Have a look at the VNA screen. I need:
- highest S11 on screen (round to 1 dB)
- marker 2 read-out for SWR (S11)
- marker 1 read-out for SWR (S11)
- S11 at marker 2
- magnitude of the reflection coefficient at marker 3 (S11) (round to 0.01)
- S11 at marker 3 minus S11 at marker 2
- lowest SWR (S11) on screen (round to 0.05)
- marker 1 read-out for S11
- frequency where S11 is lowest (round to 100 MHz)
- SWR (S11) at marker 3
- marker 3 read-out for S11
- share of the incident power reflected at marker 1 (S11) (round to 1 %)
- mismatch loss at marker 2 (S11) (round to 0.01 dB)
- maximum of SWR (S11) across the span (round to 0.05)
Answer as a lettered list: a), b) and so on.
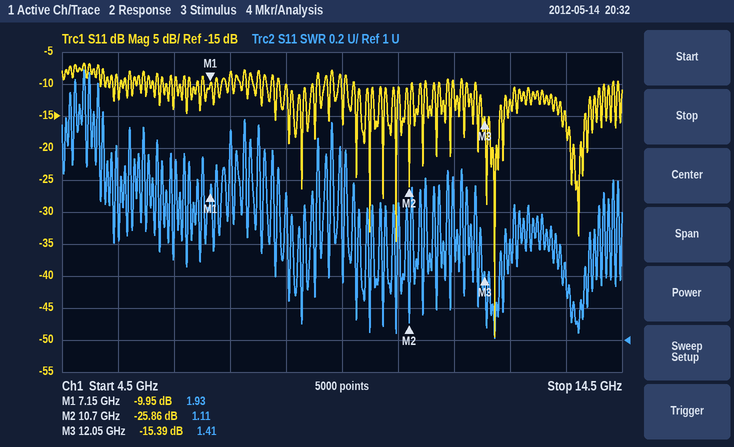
a) -7 dB
b) 1.11
c) 1.93
d) -25.86 dB
e) 0.17
f) 10.47 dB
g) 1.00
h) -9.95 dB
i) 12.2 GHz
j) 1.41
k) -15.39 dB
l) 10 %
m) 0.01 dB
n) 2.70
